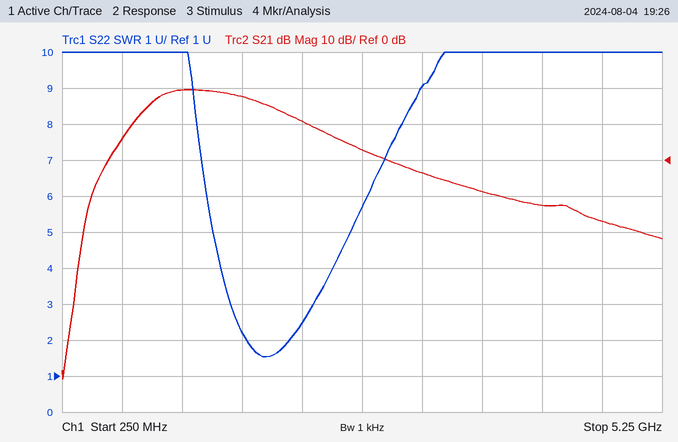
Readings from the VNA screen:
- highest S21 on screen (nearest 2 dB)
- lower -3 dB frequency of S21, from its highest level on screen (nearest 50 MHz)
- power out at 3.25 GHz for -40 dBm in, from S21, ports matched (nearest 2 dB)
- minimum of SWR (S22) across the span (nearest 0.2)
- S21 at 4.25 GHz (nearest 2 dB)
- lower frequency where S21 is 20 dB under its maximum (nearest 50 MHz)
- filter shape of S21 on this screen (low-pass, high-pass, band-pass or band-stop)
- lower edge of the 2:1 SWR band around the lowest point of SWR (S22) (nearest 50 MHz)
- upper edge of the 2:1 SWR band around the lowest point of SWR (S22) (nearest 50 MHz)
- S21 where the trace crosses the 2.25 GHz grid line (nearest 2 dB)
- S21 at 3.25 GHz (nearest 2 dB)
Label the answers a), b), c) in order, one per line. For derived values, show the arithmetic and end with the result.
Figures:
a) 20 dB
b) 1.00 GHz
c) -40 dBm + (-4 dB) = -44 dBm
d) 1.6
e) -12 dB
f) 650 MHz
g) band-pass
h) 1.80 GHz
i) 2.15 GHz
j) 10 dB
k) -4 dB
